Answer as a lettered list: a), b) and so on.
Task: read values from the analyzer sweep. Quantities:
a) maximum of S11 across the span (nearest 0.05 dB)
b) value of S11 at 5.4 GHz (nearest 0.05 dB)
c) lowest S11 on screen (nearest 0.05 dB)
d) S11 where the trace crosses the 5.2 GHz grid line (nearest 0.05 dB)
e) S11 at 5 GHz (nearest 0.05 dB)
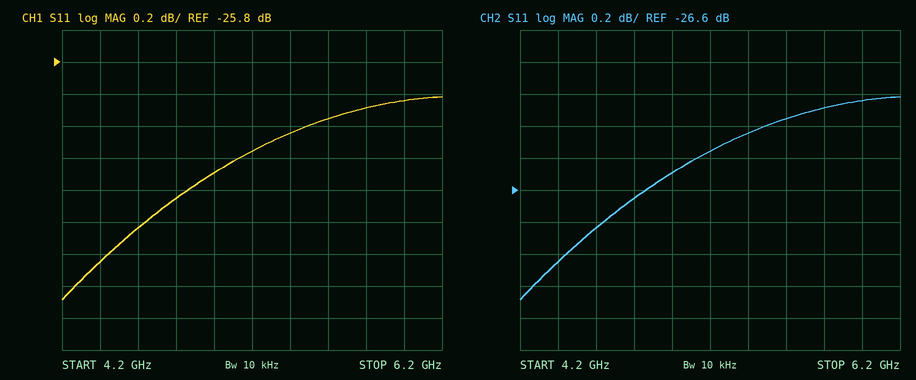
a) -26.00 dB
b) -26.25 dB
c) -27.30 dB
d) -26.35 dB
e) -26.50 dB
